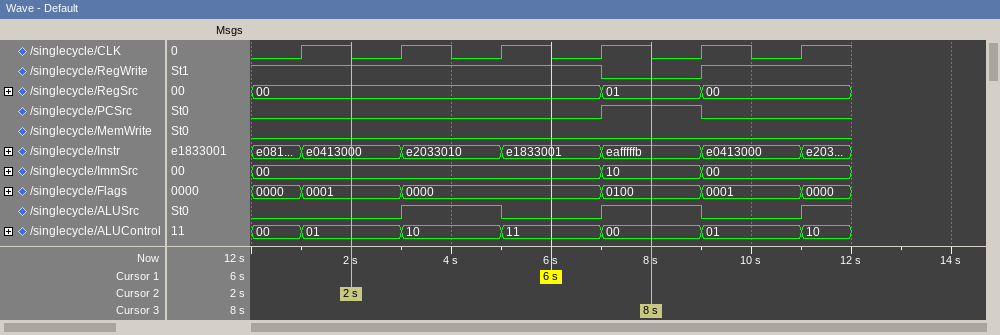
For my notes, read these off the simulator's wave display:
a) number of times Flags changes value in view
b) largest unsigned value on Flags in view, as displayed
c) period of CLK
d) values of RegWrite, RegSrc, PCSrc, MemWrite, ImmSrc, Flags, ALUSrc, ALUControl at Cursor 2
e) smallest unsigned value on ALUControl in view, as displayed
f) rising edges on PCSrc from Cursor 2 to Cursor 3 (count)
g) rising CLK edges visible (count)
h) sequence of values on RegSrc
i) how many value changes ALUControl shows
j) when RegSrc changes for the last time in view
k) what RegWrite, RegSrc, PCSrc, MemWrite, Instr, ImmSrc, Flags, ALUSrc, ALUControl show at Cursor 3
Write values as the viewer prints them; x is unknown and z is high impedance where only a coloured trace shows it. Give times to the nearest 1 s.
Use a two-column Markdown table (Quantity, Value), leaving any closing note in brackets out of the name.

| Quantity | Value |
|---|---|
| number of times Flags changes value in view | 5 |
| largest unsigned value on Flags in view, as displayed | 0100 |
| period of CLK | 2 s |
| values of RegWrite, RegSrc, PCSrc, MemWrite, ImmSrc, Flags, ALUSrc, ALUControl at Cursor 2 | RegWrite=1, RegSrc=00, PCSrc=0, MemWrite=0, ImmSrc=00, Flags=0001, ALUSrc=0, ALUControl=01 |
| smallest unsigned value on ALUControl in view, as displayed | 00 |
| rising edges on PCSrc from Cursor 2 to Cursor 3 | 1 |
| rising CLK edges visible | 6 |
| sequence of values on RegSrc | 00, 01, 00 |
| how many value changes ALUControl shows | 6 |
| when RegSrc changes for the last time in view | 9 s |
| what RegWrite, RegSrc, PCSrc, MemWrite, Instr, ImmSrc, Flags, ALUSrc, ALUControl show at Cursor 3 | RegWrite=0, RegSrc=01, PCSrc=1, MemWrite=0, Instr=eafffffb, ImmSrc=10, Flags=0100, ALUSrc=1, ALUControl=00 |
